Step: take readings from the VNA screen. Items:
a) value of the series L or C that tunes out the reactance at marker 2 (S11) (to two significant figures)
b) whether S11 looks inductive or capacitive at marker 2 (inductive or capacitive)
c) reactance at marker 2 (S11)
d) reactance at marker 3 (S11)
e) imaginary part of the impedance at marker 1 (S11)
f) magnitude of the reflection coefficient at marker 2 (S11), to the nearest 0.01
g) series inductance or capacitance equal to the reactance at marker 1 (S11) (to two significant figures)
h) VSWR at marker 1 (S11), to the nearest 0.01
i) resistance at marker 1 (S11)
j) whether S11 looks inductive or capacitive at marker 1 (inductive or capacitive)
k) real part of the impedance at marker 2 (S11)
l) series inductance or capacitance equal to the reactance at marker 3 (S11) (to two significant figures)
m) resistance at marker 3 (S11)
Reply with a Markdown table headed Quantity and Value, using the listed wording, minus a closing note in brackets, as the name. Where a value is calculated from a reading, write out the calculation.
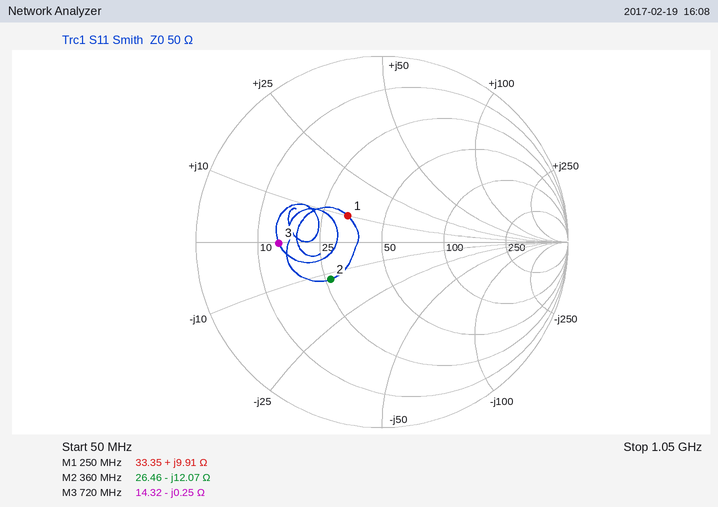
| Quantity | Value |
|---|---|
| value of the series L or C that tunes out the reactance at marker 2 (S11) | L = 12.07 Ω/(2π × 360 MHz) ≈ 5.3 nH |
| whether S11 looks inductive or capacitive at marker 2 | capacitive |
| reactance at marker 2 | -12.07 Ω |
| reactance at marker 3 | -0.25 Ω |
| imaginary part of the impedance at marker 1 | +9.91 Ω |
| magnitude of the reflection coefficient at marker 2 (S11), to the nearest 0.01 | 0.34 |
| series inductance or capacitance equal to the reactance at marker 1 (S11) | L = 9.91 Ω/(2π × 250 MHz) ≈ 6.3 nH |
| VSWR at marker 1 (S11), to the nearest 0.01 | 1.60 |
| resistance at marker 1 | 33.35 Ω |
| whether S11 looks inductive or capacitive at marker 1 | inductive |
| real part of the impedance at marker 2 | 26.46 Ω |
| series inductance or capacitance equal to the reactance at marker 3 (S11) | C = 1/(2π × 720 MHz × 0.25 Ω) ≈ 884 pF, so 880 pF to two significant figures |
| resistance at marker 3 | 14.32 Ω |
